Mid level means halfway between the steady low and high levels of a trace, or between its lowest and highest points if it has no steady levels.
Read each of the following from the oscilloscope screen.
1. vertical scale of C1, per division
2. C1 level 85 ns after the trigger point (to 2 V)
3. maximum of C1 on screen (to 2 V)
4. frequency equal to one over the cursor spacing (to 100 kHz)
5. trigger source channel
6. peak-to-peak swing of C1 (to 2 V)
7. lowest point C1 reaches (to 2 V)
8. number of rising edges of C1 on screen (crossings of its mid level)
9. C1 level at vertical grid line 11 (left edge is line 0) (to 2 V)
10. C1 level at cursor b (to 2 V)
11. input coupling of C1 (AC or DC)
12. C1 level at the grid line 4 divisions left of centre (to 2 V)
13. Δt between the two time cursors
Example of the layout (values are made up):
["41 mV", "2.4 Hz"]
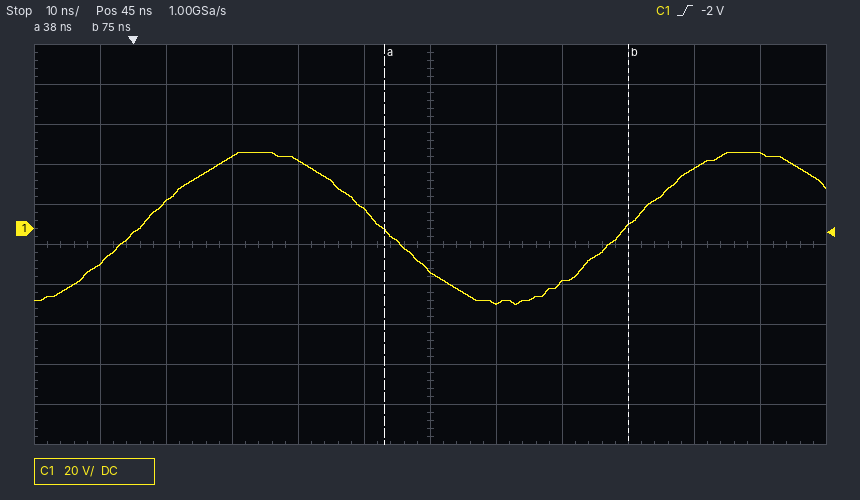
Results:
["20 V", "30 V", "38 V", "27.0 MHz", "C1", "76 V", "-38 V", "2", "38 V", "2 V", "DC", "14 V", "37 ns"]
